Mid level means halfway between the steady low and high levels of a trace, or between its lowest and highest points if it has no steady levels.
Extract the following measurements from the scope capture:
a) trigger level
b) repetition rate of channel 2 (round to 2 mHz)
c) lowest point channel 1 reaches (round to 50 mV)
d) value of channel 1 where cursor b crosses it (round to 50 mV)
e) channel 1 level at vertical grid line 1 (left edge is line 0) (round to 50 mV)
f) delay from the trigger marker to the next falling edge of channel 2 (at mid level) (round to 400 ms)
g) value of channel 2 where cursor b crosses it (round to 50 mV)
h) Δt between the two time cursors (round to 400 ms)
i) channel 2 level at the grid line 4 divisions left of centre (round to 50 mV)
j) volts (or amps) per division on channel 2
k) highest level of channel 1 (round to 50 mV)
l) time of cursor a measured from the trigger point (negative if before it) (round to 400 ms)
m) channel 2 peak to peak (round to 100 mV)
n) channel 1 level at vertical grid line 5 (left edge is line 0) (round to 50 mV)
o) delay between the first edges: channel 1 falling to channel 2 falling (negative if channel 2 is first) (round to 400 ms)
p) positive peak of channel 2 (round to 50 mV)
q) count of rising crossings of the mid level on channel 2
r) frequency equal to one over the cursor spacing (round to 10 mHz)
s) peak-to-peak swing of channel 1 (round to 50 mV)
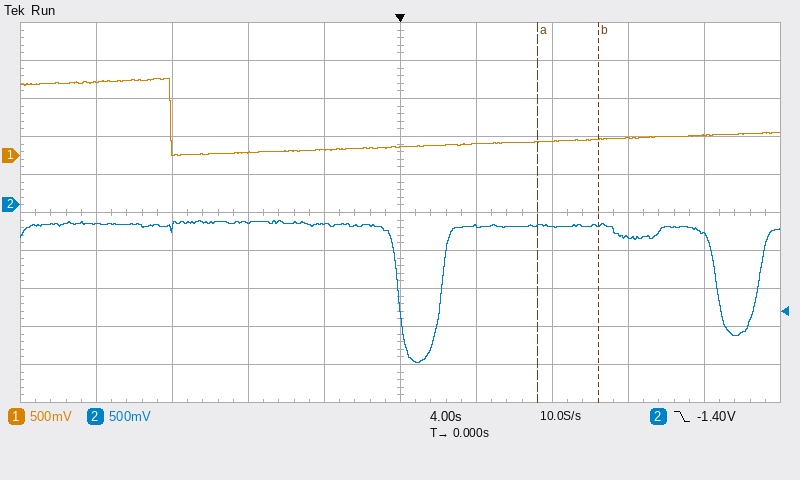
-1.40 V
60 mHz
0 mV
200 mV
950 mV
16.8 s
-250 mV
3.2 s
-250 mV
500 mV
1.00 V
+7.2 s
1.90 V
100 mV
+12.0 s
-200 mV
2
310 mHz
1.00 V
